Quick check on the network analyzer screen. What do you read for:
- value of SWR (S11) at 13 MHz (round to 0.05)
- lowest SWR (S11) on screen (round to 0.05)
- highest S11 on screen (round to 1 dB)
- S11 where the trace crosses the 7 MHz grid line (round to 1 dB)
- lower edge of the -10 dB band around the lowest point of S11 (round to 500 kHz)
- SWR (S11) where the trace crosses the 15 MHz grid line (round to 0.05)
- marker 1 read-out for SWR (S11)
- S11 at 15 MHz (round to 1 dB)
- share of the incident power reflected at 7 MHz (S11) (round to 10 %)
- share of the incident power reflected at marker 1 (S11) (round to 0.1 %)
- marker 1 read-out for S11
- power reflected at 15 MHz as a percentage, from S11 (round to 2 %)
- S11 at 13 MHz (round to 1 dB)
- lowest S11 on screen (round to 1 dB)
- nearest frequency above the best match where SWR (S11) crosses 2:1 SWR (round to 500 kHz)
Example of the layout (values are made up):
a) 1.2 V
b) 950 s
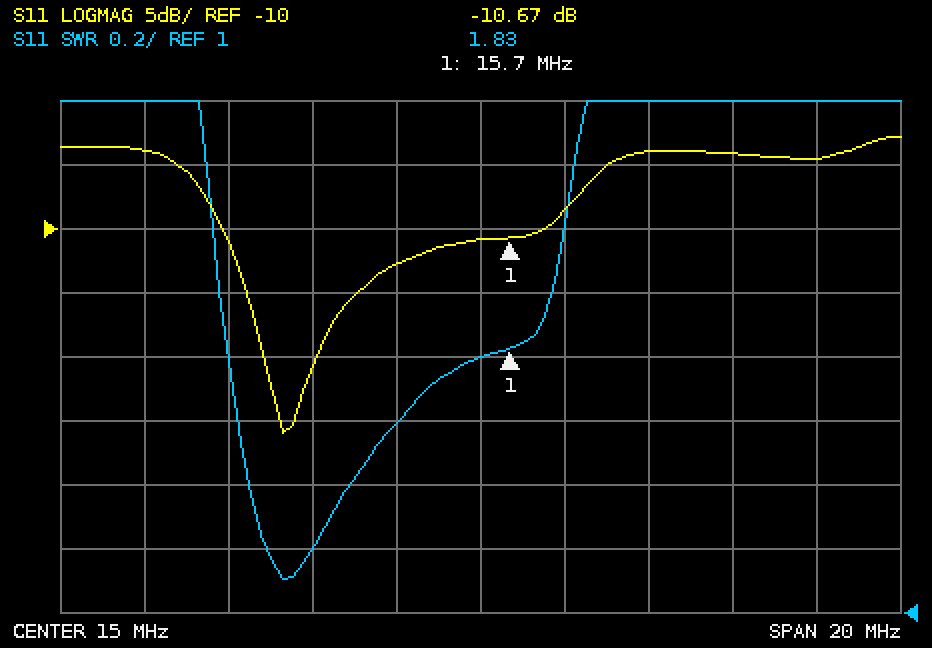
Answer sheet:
a) 1.60
b) 1.10
c) -3 dB
d) -4 dB
e) 9.0 MHz
f) 1.80
g) 1.83
h) -11 dB
i) 40 %
j) 8.6 %
k) -10.67 dB
l) 8 %
m) -13 dB
n) -26 dB
o) 16.5 MHz
